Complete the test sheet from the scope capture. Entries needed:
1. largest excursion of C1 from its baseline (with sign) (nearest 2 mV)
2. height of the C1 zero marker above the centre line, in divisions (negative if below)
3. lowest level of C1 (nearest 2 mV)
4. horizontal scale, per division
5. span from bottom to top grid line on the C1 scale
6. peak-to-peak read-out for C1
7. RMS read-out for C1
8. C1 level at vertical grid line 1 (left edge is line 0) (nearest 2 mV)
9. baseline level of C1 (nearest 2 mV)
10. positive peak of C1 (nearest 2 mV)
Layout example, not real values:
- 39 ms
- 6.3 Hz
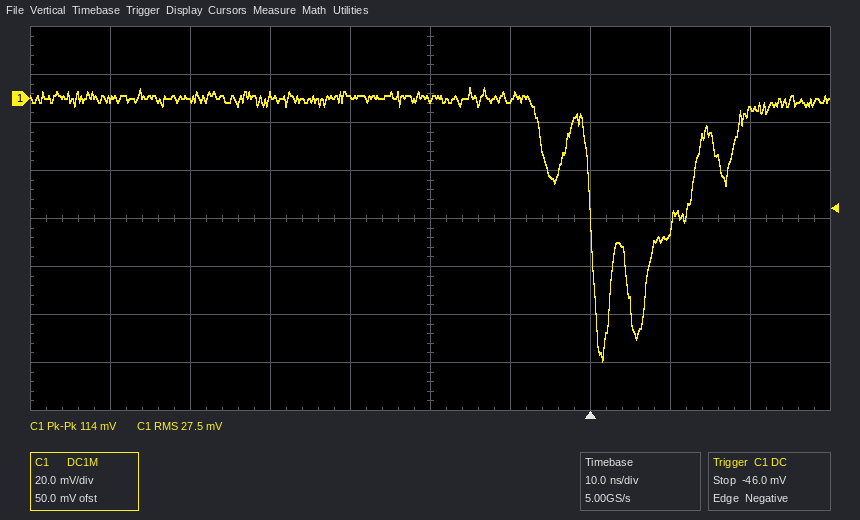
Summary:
- -110 mV
- +2.5 div
- -110 mV
- 10 ns
- 160 mV
- 114 mV
- 27.5 mV
- 0 mV
- 0 mV
- 4 mV
